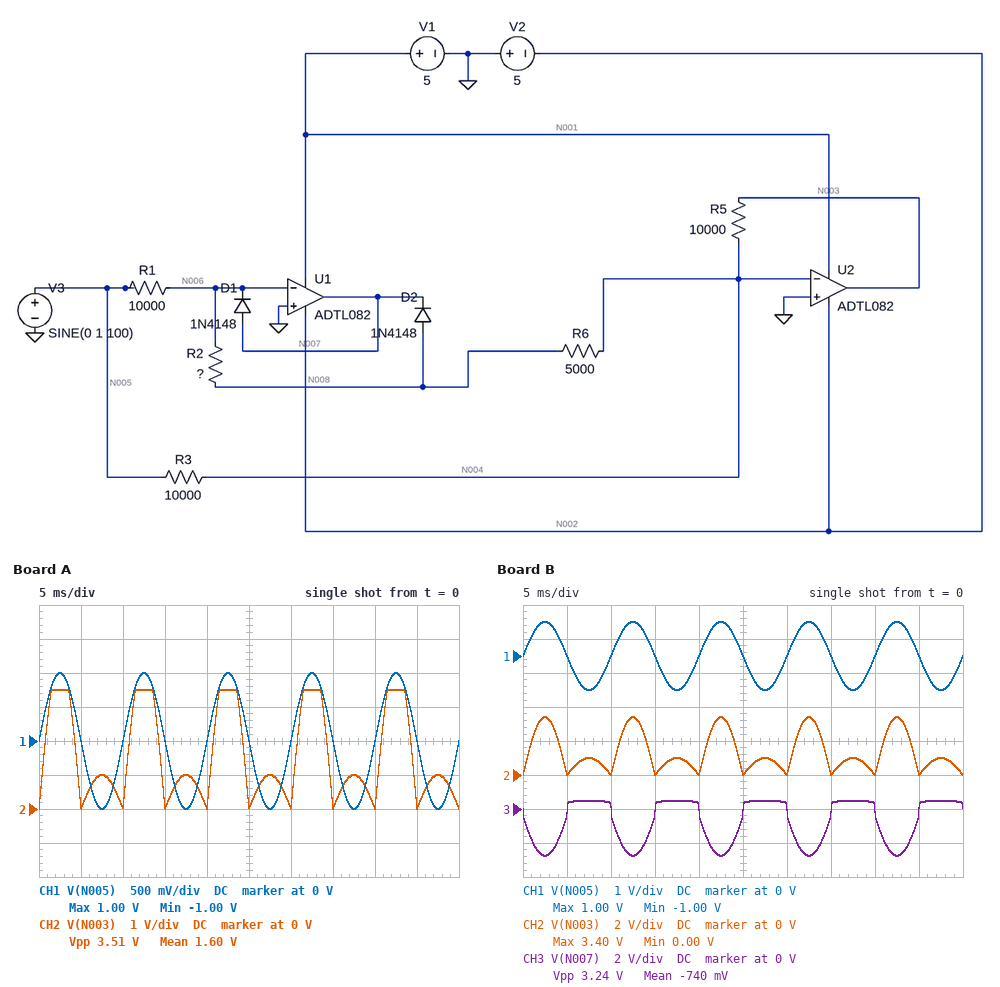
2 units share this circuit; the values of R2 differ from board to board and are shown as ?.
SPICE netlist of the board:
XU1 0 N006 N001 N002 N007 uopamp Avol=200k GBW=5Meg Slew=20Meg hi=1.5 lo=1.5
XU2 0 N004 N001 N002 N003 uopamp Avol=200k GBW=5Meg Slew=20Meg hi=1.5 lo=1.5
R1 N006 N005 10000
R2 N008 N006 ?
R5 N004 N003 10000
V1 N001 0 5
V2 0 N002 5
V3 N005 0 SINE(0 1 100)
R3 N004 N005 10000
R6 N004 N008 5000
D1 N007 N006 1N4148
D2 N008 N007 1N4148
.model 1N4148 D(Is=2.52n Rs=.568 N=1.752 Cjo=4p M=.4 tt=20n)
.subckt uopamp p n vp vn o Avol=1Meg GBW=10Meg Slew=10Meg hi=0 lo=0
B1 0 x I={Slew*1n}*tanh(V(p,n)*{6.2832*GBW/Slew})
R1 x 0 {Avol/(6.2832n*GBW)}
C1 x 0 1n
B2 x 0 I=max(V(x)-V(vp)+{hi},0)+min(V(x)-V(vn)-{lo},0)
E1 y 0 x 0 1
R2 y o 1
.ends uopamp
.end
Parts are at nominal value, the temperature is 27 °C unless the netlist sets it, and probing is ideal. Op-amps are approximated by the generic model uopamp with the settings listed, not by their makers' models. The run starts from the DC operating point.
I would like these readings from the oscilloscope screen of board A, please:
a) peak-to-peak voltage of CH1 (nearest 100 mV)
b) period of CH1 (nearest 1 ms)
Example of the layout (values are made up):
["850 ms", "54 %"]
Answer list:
["2.0 V", "10 ms"]
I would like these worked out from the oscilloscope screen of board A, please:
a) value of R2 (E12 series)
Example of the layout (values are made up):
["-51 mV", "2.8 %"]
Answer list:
["27 kΩ"]
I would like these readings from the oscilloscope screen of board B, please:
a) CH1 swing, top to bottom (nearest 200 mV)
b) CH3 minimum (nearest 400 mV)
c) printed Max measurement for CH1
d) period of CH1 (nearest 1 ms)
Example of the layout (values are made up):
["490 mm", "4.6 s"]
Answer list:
["2.0 V", "-2.8 V", "1.00 V", "10 ms"]
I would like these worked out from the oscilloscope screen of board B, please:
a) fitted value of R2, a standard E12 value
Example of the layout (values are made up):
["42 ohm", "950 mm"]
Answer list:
["22 kΩ"]
